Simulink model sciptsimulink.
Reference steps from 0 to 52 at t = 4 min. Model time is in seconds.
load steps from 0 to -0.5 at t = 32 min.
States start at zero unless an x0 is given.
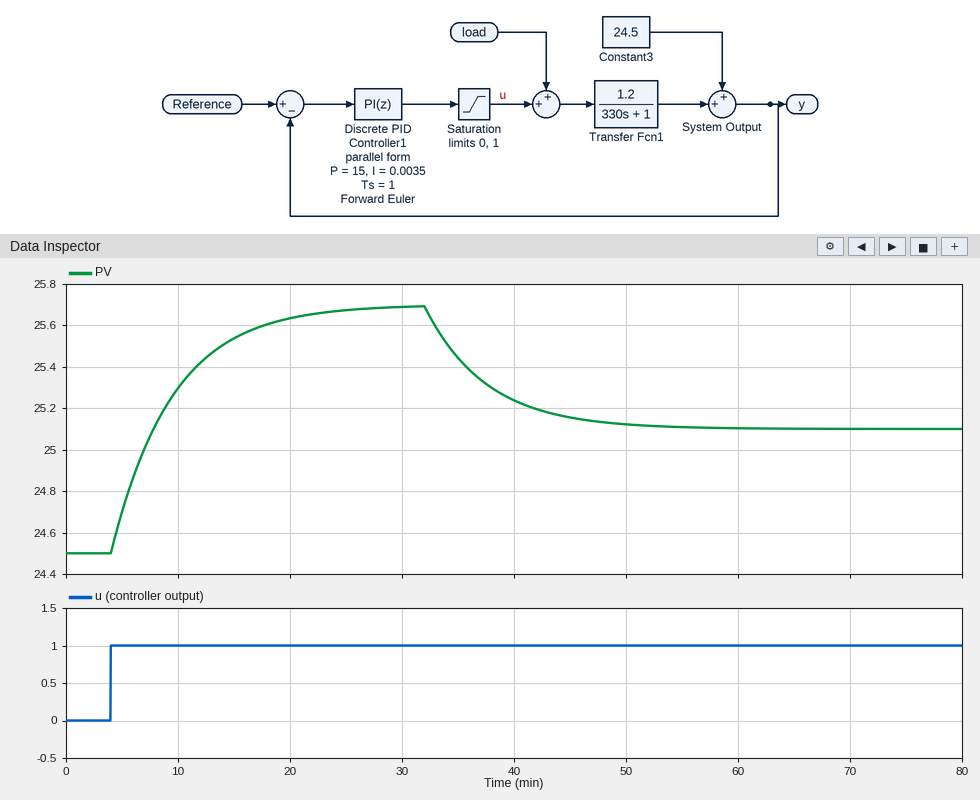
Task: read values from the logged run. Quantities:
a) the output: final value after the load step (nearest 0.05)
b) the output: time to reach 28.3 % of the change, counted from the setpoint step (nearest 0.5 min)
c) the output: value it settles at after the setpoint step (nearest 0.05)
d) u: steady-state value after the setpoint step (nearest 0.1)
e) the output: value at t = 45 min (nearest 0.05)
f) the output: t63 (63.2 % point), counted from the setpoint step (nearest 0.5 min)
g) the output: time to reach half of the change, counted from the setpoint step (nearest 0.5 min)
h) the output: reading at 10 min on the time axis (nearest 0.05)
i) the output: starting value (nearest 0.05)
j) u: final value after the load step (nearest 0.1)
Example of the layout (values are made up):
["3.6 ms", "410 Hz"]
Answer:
["25.10", "2.0 min", "25.70", "1.0", "25.15", "5.5 min", "4.0 min", "25.30", "24.50", "1.0"]
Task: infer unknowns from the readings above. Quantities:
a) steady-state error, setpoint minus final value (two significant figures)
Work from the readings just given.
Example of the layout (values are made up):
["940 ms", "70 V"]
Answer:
["26"]
